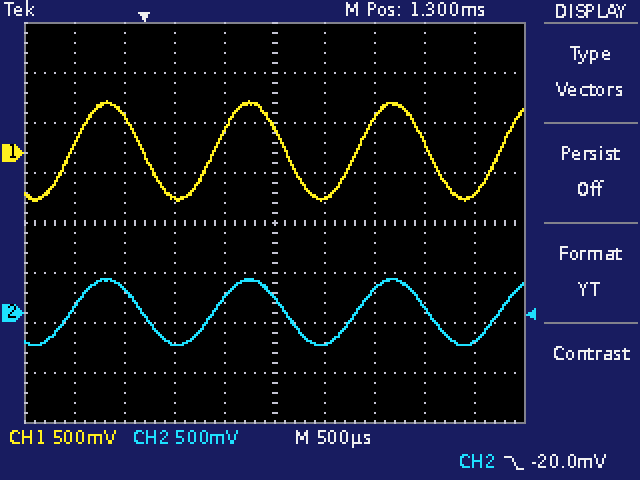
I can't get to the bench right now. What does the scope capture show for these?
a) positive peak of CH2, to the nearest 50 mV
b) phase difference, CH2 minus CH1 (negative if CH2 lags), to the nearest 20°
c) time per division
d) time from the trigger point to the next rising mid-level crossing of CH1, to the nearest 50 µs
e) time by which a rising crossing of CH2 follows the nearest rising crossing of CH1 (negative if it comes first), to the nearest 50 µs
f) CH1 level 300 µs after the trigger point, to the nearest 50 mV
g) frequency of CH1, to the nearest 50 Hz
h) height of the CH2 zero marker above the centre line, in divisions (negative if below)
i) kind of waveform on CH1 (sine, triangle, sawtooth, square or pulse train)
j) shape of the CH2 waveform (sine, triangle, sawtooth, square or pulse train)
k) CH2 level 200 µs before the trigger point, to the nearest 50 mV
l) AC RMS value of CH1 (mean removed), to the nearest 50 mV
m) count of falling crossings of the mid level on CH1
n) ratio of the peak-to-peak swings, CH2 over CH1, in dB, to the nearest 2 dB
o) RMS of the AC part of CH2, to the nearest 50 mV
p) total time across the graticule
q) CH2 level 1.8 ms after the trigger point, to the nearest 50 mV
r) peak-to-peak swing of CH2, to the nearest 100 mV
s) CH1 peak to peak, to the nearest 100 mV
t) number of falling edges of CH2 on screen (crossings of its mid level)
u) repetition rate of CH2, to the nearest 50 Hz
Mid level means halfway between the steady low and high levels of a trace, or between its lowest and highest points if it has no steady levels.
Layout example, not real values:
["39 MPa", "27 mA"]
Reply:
["350 mV", "0°", "500 µs", "700 µs", "0 µs", "-450 mV", "700 Hz", "-1.8 div", "sine", "sine", "250 mV", "350 mV", "3", "-4 dB", "250 mV", "5 ms", "-300 mV", "700 mV", "1.00 V", "3", "700 Hz"]
